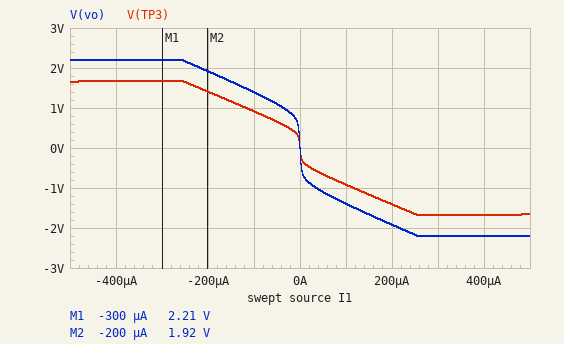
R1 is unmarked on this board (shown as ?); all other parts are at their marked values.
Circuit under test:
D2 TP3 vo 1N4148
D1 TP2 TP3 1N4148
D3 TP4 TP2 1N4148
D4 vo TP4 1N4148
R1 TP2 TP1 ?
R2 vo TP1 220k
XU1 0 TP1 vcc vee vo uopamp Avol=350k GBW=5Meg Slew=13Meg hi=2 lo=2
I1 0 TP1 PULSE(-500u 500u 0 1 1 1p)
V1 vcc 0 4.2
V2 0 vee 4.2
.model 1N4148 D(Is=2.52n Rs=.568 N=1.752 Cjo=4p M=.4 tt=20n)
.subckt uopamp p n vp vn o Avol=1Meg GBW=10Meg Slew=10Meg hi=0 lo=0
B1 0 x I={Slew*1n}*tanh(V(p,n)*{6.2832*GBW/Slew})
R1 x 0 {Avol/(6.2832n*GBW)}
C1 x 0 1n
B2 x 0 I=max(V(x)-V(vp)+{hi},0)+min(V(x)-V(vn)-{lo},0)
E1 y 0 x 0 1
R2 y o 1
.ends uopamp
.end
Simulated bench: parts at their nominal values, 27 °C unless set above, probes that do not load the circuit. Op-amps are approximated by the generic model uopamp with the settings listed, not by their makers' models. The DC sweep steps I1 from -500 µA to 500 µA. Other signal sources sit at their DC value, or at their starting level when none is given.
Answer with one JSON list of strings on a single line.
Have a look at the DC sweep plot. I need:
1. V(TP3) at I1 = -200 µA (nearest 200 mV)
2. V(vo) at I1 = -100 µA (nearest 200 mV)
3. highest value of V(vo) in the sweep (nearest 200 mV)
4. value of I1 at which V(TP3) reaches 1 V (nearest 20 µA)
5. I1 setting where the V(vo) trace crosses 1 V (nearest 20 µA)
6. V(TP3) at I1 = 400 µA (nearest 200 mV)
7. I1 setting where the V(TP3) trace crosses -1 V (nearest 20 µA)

["1.4 V", "1.4 V", "2.2 V", "-120 µA", "-40 µA", "-1.6 V", "120 µA"]
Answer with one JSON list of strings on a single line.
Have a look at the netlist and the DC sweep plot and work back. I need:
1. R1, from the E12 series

["4.7 kΩ"]
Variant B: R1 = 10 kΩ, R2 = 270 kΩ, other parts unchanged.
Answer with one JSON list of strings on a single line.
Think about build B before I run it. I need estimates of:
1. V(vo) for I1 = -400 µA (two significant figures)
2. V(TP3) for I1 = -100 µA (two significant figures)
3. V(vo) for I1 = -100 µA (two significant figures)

["2.2 V", "1.4 V", "1.9 V"]
